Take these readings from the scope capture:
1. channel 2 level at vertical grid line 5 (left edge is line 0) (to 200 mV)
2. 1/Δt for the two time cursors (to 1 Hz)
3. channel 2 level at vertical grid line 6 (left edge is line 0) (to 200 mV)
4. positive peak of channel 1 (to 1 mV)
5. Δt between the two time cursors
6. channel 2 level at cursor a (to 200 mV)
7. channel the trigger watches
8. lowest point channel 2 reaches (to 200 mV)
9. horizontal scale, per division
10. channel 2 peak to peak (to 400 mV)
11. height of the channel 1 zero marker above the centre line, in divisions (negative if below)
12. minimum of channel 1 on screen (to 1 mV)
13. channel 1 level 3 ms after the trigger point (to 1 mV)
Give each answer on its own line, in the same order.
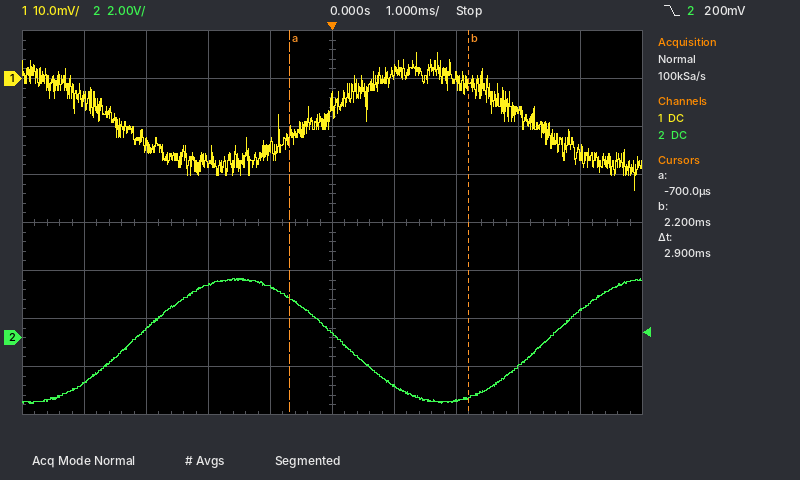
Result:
200 mV
345 Hz
-2.0 V
5 mV
2.9 ms
1.6 V
channel 2
-2.8 V
1 ms
5.2 V
+3.0 div
-23 mV
-7 mV
